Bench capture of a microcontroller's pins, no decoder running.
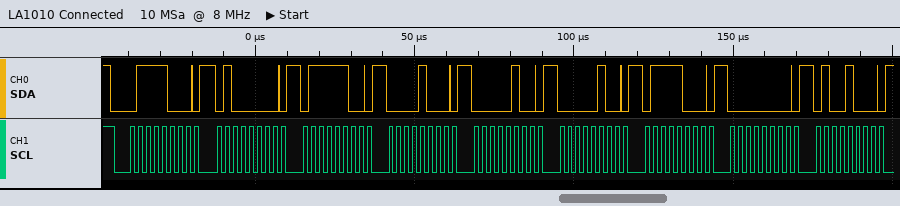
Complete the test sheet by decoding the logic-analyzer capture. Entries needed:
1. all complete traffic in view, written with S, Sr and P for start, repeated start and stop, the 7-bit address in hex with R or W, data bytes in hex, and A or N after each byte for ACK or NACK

S 3CW A 40 A 7C A 08 A 04 A 04 A 78 A 00 A 48 A
